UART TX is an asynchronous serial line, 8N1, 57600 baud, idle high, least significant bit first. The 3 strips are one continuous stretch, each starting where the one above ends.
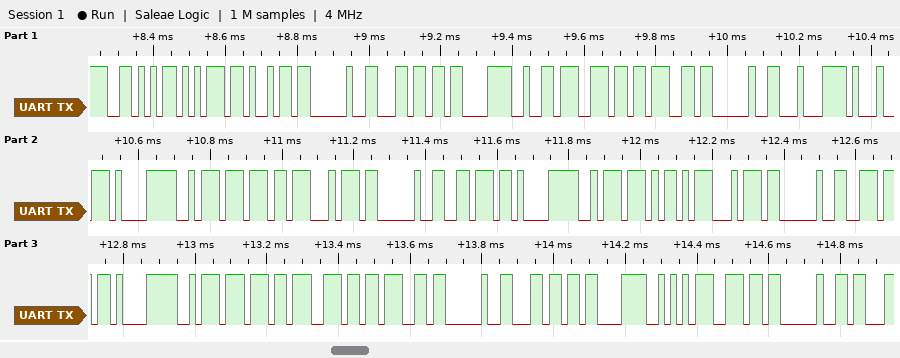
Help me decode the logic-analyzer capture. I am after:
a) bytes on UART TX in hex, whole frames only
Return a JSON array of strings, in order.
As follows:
["0x56 0x75 0x69 0x20 0x6C 0xC3 0xB2 0x6E 0x67 0x20 0xC4 0x91 0xE1 0xBA 0xB7 0x74 0x20 0x76 0xE1 0xBA 0xAD 0x74 0x20 0x6E 0xE1 0xBA 0xB7 0x6E 0x67 0x20 0x6C 0xC3 0xAA 0x6E 0x20"]
